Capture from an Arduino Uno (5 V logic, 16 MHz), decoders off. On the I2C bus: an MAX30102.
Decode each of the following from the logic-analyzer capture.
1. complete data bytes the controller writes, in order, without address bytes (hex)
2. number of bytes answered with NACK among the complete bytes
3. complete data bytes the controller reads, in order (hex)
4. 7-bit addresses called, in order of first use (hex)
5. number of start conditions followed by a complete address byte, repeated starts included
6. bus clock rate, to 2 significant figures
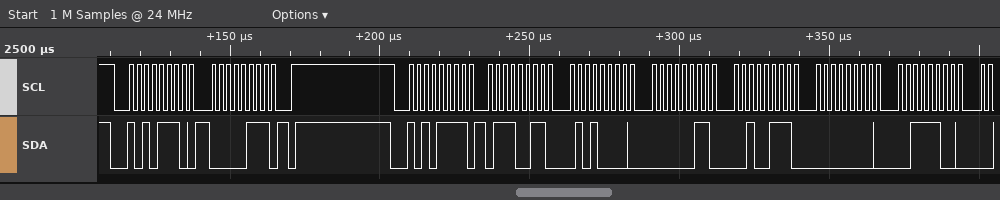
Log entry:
07
0
73 50 03 27 00 3C
0x57
2
400 kHz
